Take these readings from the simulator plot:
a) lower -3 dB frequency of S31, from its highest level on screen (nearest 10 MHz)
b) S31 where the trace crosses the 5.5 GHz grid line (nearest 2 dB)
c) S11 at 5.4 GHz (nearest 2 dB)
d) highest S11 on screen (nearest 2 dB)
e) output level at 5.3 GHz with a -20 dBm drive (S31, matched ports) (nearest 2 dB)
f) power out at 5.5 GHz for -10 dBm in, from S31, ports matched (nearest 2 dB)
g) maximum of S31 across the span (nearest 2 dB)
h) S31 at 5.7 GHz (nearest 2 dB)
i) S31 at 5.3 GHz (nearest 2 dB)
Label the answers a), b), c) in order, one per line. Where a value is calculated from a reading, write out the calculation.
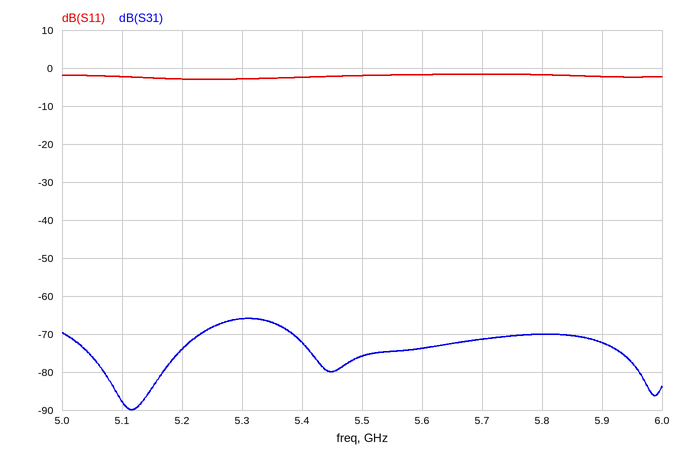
a) 5.24 GHz
b) -76 dB
c) -2 dB
d) -2 dB
e) -20 dBm + (-66 dB) = -86 dBm
f) -10 dBm + (-76 dB) = -86 dBm
g) -66 dB
h) -72 dB
i) -66 dB
